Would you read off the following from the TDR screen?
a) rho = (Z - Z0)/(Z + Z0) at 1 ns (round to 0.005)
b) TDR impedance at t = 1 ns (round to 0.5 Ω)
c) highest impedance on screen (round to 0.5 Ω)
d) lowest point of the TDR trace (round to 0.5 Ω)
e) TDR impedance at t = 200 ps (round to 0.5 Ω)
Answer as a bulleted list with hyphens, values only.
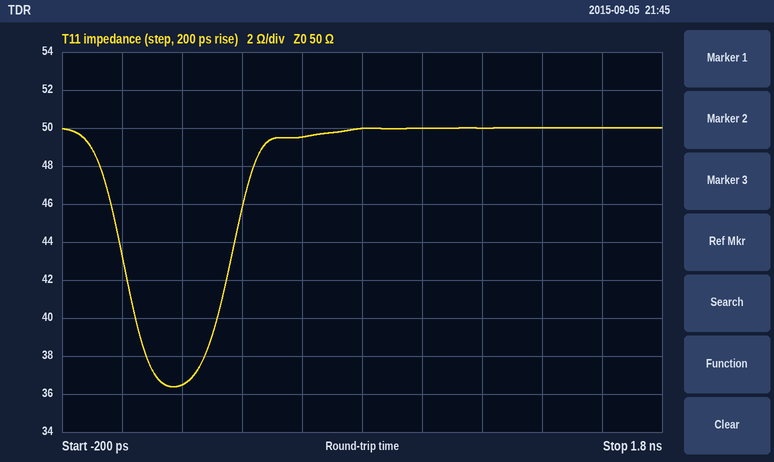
- 0.000
- 50.0 Ω
- 50.0 Ω
- 36.5 Ω
- 36.5 Ω
